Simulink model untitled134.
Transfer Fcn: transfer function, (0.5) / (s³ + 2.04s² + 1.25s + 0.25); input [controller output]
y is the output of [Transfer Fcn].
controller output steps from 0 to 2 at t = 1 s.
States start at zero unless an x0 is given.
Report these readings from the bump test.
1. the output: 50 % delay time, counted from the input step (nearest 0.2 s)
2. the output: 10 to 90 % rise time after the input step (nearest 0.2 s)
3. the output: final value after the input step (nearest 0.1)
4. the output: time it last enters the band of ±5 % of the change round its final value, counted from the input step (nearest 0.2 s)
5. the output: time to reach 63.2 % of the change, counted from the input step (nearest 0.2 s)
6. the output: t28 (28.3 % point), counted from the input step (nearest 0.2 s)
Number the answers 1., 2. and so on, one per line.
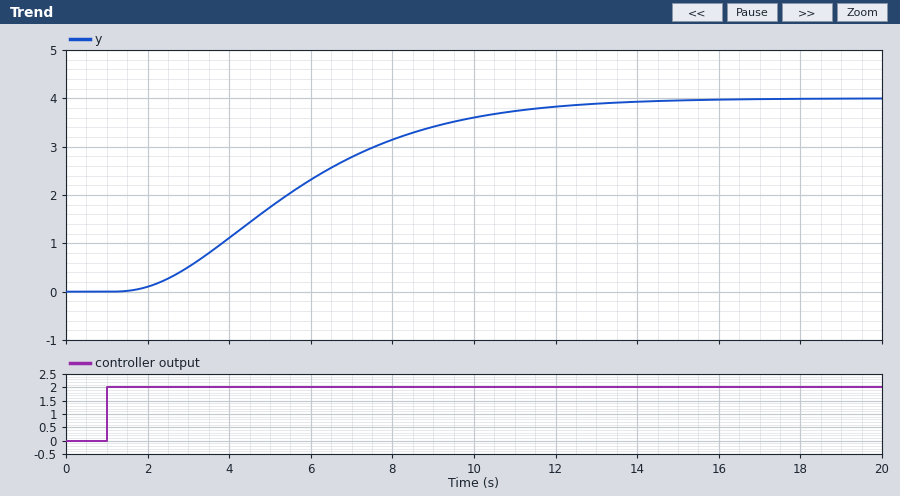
1. 4.4 s
2. 7.2 s
3. 4.0
4. 10.6 s
5. 5.4 s
6. 3.0 s
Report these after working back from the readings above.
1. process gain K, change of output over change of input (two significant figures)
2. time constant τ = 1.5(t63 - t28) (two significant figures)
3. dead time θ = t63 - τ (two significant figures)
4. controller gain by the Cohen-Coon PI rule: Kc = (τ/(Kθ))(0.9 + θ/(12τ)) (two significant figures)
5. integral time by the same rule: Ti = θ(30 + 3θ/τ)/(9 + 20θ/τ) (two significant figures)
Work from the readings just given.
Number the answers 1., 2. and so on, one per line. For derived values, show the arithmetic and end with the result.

1. (4 - 0) / 2 = 2.0
2. 1.5 × (5.4 - 3) = 3.6 s
3. 5.4 - 3.6 = 1.8 s
4. 3.6 / (2 × 1.8) × (0.9 + 1.8 / (12 × 3.6)) = 0.94
5. 1.8 × (30 + 3 × 1.8 / 3.6) / (9 + 20 × 1.8 / 3.6) = 3.0 s
